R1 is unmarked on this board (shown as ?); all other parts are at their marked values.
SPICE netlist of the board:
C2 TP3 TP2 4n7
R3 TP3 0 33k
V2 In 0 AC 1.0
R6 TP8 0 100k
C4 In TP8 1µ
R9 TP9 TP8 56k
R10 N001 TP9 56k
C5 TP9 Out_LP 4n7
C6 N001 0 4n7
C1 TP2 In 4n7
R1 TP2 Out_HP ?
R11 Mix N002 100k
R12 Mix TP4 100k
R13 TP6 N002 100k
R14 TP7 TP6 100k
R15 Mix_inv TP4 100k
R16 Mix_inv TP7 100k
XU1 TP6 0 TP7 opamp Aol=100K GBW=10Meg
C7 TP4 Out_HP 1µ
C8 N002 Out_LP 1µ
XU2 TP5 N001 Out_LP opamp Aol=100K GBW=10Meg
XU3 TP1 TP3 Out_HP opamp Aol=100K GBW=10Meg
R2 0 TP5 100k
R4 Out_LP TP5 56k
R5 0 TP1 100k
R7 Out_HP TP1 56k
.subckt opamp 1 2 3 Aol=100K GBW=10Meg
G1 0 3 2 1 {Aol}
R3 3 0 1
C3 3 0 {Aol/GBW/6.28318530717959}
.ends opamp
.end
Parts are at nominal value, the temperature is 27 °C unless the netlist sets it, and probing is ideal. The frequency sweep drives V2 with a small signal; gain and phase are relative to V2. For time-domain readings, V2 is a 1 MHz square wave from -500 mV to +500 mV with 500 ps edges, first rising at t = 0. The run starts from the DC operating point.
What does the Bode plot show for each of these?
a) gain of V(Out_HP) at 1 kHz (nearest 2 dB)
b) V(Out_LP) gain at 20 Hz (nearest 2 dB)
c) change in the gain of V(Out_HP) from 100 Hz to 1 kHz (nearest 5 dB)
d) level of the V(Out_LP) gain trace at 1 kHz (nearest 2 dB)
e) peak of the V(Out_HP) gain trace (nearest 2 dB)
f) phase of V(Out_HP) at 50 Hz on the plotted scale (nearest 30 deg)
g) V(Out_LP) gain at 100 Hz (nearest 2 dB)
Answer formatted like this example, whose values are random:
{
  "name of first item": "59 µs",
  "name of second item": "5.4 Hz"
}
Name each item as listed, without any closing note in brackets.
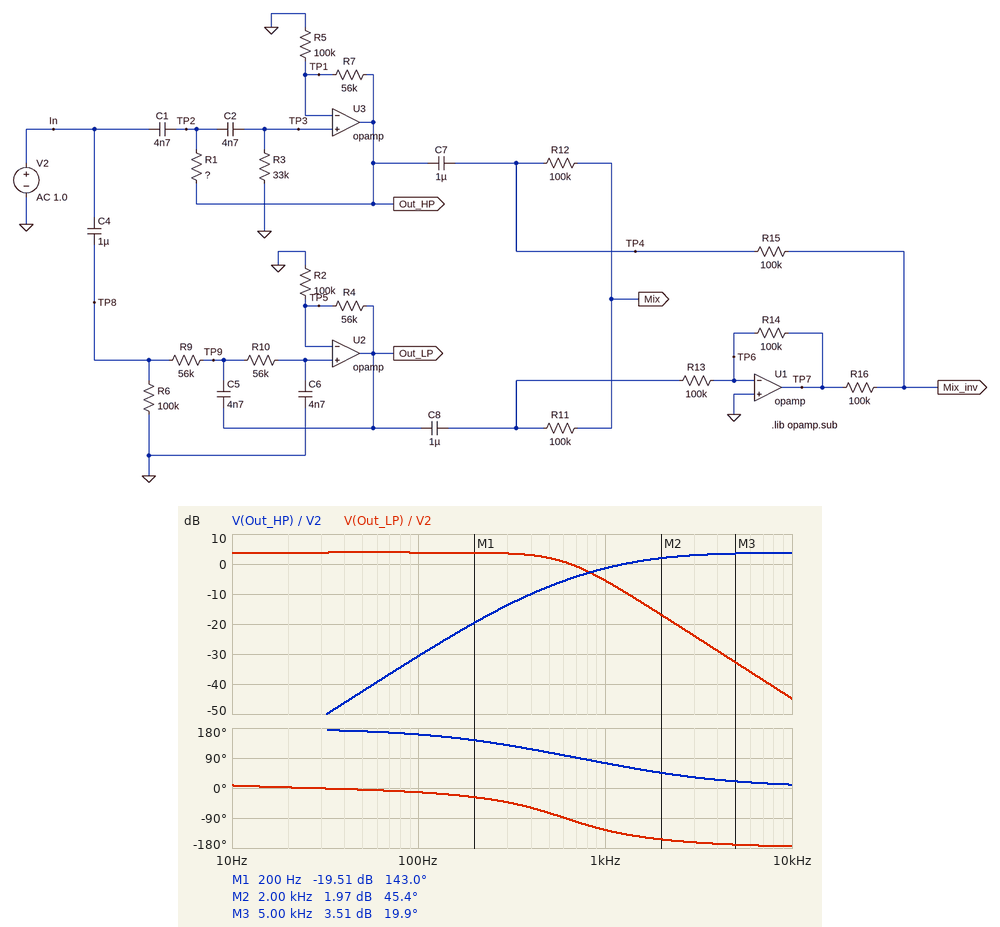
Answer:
{
  "gain of V(Out_HP) at 1 kHz": "-2 dB",
  "V(Out_LP) gain at 20 Hz": "4 dB",
  "change in the gain of V(Out_HP) from 100 Hz to 1 kHz": "30 dB",
  "level of the V(Out_LP) gain trace at 1 kHz": "-6 dB",
  "peak of the V(Out_HP) gain trace": "4 dB",
  "phase of V(Out_HP) at 50 Hz on the plotted scale": "180 deg",
  "V(Out_LP) gain at 100 Hz": "4 dB"
}
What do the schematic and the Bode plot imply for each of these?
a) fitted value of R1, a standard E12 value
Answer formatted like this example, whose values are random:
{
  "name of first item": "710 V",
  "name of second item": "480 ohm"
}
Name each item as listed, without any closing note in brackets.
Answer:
{
  "fitted value of R1, a standard E12 value": "68 kΩ"
}
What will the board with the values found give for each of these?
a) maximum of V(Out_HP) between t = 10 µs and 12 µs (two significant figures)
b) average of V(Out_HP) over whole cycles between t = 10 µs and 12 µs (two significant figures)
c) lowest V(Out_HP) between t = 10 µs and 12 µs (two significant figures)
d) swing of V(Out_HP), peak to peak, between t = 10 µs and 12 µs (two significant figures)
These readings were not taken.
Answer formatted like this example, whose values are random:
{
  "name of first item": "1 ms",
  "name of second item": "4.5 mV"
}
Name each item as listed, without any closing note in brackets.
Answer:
{
  "maximum of V(Out_HP) between t = 10 µs and 12 µs": "1.5 V",
  "average of V(Out_HP) over whole cycles between t = 10 µs and 12 µs": "690 mV",
  "lowest V(Out_HP) between t = 10 µs and 12 µs": "-99 mV",
  "swing of V(Out_HP), peak to peak, between t = 10 µs and 12 µs": "1.6 V"
}
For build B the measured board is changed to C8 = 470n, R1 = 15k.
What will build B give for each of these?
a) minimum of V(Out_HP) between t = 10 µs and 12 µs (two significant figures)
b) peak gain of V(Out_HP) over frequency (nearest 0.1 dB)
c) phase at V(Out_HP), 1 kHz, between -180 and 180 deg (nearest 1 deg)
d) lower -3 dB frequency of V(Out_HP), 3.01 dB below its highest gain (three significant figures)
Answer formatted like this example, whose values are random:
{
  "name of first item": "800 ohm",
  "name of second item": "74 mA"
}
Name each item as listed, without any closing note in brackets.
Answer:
{
  "minimum of V(Out_HP) between t = 10 µs and 12 µs": "-50 mV",
  "peak gain of V(Out_HP) over frequency": "9.9 dB",
  "phase at V(Out_HP), 1 kHz, between -180 and 180 deg": "149 deg",
  "lower -3 dB frequency of V(Out_HP), 3.01 dB below its highest gain": "1.30 kHz"
}
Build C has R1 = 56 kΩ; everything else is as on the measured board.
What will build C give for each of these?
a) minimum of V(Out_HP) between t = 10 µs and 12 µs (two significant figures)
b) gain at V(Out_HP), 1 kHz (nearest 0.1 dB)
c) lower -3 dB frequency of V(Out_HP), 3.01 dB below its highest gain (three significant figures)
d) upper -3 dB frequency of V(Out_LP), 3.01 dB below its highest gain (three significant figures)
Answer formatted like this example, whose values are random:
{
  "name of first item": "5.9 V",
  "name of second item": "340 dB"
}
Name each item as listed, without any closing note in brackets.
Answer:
{
  "minimum of V(Out_HP) between t = 10 µs and 12 µs": "-96 mV",
  "gain at V(Out_HP), 1 kHz": "-1.0 dB",
  "lower -3 dB frequency of V(Out_HP), 3.01 dB below its highest gain": "1.38 kHz",
  "upper -3 dB frequency of V(Out_LP), 3.01 dB below its highest gain": "593 Hz"
}
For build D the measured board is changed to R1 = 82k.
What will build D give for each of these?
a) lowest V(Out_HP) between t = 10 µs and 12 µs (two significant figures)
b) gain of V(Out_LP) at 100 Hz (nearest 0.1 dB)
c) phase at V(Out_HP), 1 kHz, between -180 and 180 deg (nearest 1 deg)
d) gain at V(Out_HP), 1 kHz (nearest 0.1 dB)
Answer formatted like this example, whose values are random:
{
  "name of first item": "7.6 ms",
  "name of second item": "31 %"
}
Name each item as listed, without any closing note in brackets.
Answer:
{
  "lowest V(Out_HP) between t = 10 µs and 12 µs": "-100 mV",
  "gain of V(Out_LP) at 100 Hz": "3.8 dB",
  "phase at V(Out_HP), 1 kHz, between -180 and 180 deg": "72 deg",
  "gain at V(Out_HP), 1 kHz": "-1.8 dB"
}
